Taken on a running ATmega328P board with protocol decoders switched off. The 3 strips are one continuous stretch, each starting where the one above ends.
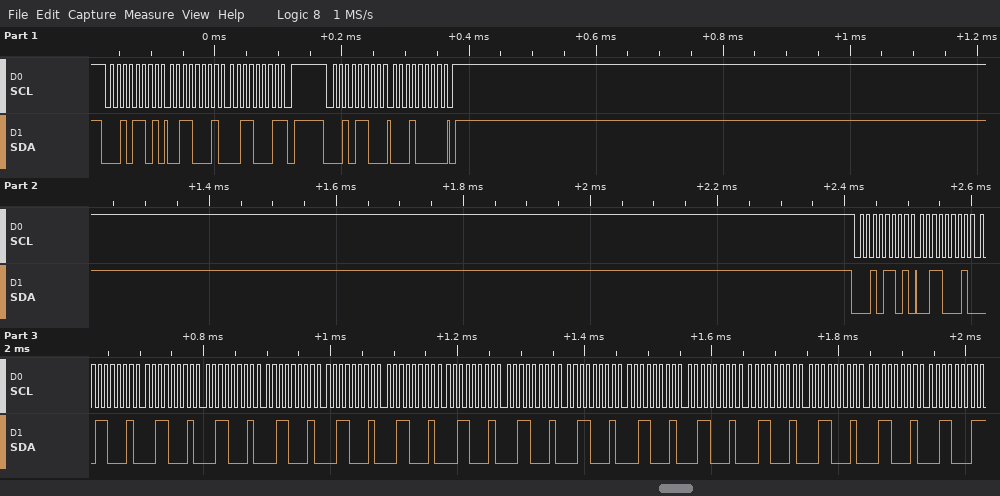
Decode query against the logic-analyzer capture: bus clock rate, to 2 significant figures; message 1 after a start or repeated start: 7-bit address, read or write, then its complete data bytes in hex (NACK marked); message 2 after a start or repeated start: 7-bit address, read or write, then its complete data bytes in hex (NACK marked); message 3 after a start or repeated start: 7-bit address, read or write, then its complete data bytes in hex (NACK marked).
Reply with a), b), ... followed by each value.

a) 100 kHz
b) 0x16 read: 31 31 NACK
c) 0x16 write: 10
d) 0x16 read: 31 31 31 31 31 31 31 31 31 31 31 31 31 31 31 31 NACK
